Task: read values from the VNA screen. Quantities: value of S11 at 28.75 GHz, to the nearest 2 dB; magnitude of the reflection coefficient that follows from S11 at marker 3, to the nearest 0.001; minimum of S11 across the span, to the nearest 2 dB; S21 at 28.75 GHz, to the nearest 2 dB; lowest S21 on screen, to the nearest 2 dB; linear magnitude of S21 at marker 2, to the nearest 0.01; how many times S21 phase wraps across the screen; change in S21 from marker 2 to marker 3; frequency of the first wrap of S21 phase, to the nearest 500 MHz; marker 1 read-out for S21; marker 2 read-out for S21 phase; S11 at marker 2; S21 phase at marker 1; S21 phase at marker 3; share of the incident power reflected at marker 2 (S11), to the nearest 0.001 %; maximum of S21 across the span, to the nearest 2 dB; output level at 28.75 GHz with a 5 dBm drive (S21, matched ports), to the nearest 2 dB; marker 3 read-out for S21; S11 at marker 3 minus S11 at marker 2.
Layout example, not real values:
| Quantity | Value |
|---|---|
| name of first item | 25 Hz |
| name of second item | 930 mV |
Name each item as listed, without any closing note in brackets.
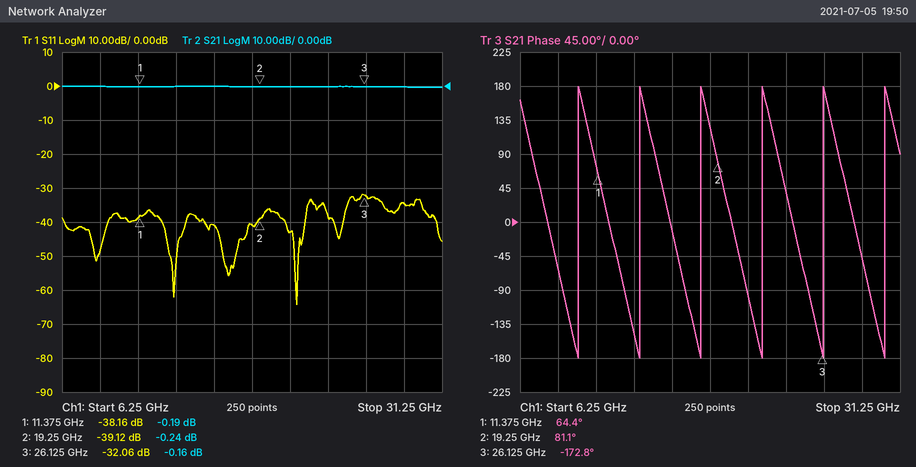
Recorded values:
| Quantity | Value |
|---|---|
| value of S11 at 28.75 GHz, to the nearest 2 dB | -34 dB |
| magnitude of the reflection coefficient that follows from S11 at marker 3, to the nearest 0.001 | 0.025 |
| minimum of S11 across the span, to the nearest 2 dB | -64 dB |
| S21 at 28.75 GHz, to the nearest 2 dB | 0 dB |
| lowest S21 on screen, to the nearest 2 dB | 0 dB |
| linear magnitude of S21 at marker 2, to the nearest 0.01 | 0.97 |
| how many times S21 phase wraps across the screen | 6 |
| change in S21 from marker 2 to marker 3 | 0.08 dB |
| frequency of the first wrap of S21 phase, to the nearest 500 MHz | 10.0 GHz |
| marker 1 read-out for S21 | -0.19 dB |
| marker 2 read-out for S21 phase | 81.1° |
| S11 at marker 2 | -39.12 dB |
| S21 phase at marker 1 | 64.4° |
| S21 phase at marker 3 | -172.8° |
| share of the incident power reflected at marker 2 (S11), to the nearest 0.001 % | 0.012 % |
| maximum of S21 across the span, to the nearest 2 dB | 0 dB |
| output level at 28.75 GHz with a 5 dBm drive (S21, matched ports), to the nearest 2 dB | 4 dBm |
| marker 3 read-out for S21 | -0.16 dB |
| S11 at marker 3 minus S11 at marker 2 | 7.06 dB |
